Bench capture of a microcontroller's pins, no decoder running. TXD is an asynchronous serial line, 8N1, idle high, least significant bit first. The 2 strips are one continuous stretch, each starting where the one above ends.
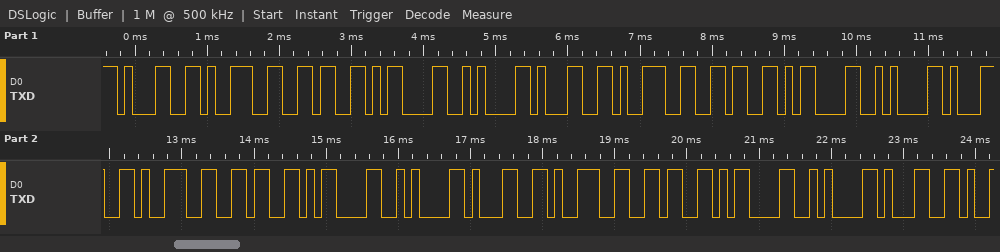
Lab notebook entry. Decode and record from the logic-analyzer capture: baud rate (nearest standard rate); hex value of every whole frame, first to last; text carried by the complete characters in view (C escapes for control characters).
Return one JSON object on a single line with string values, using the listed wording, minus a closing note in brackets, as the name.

{"baud rate": "9600 baud", "hex value of every whole frame, first to last": "31 39 36 0D 0A 31 39 36 0D 0A 31 39 36 0D 0A 31 39 36 0D 0A 31", "text carried by the complete characters in view": "\"196\\r\\n196\\r\\n196\\r\\n196\\r\\n1\""}
